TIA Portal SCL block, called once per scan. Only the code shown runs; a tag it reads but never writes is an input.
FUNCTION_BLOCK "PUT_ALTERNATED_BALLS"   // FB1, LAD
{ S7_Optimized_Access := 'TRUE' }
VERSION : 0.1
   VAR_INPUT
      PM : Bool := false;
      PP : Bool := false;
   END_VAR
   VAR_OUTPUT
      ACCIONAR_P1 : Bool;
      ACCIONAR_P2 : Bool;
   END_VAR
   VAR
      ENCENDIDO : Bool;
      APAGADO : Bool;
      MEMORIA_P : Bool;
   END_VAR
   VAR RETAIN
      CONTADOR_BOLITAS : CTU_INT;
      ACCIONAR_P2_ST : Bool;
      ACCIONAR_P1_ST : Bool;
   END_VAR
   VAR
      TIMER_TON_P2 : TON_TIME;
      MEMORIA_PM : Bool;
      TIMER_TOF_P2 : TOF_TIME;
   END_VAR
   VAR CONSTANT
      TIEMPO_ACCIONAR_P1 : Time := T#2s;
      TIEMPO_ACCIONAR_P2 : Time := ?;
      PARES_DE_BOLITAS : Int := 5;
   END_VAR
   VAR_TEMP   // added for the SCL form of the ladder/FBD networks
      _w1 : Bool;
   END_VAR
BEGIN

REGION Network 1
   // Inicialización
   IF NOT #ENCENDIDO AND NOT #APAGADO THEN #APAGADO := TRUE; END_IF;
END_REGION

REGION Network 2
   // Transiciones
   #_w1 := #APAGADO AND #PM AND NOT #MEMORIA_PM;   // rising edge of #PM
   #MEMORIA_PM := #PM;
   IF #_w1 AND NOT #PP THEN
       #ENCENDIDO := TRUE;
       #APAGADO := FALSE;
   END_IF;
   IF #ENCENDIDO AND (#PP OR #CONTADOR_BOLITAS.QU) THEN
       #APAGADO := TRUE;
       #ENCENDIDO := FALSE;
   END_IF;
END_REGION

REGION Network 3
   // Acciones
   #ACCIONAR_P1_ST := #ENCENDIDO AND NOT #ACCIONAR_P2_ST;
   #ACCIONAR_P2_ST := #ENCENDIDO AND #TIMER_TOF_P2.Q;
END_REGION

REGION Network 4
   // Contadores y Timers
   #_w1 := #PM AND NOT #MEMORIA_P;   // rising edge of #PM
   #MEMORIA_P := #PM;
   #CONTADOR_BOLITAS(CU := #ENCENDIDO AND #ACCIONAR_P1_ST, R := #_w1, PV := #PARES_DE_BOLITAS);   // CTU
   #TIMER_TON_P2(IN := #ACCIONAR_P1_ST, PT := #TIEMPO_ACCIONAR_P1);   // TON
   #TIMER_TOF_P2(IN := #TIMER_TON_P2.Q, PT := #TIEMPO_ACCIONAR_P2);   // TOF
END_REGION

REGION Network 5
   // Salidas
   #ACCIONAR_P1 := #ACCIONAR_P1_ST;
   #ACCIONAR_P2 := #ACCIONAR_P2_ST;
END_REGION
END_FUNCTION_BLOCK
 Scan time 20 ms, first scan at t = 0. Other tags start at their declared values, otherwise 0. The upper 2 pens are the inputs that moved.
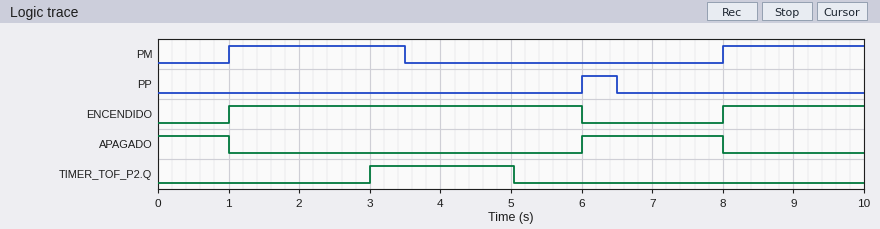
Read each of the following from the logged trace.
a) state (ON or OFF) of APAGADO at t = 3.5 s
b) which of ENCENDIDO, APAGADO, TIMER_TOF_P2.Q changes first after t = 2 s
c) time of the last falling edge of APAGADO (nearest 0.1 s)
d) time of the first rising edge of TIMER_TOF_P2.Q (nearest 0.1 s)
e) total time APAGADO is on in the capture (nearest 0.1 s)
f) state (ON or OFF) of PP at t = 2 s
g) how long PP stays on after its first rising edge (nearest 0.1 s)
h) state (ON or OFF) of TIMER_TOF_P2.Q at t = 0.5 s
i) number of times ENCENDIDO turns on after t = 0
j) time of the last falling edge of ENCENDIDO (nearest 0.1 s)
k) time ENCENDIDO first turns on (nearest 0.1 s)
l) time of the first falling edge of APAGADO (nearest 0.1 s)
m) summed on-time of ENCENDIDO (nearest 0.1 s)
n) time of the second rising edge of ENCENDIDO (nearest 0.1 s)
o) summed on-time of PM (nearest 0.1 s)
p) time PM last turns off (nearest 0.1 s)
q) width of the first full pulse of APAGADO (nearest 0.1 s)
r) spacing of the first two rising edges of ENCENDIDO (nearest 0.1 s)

OFF
TIMER_TOF_P2.Q
8.0 s
3.0 s
3.0 s
OFF
0.5 s
OFF
2
6.0 s
1.0 s
1.0 s
7.0 s
8.0 s
4.5 s
3.5 s
2.0 s
7.0 s
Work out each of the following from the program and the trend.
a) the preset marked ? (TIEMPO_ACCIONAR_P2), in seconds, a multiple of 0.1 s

2.0 s
